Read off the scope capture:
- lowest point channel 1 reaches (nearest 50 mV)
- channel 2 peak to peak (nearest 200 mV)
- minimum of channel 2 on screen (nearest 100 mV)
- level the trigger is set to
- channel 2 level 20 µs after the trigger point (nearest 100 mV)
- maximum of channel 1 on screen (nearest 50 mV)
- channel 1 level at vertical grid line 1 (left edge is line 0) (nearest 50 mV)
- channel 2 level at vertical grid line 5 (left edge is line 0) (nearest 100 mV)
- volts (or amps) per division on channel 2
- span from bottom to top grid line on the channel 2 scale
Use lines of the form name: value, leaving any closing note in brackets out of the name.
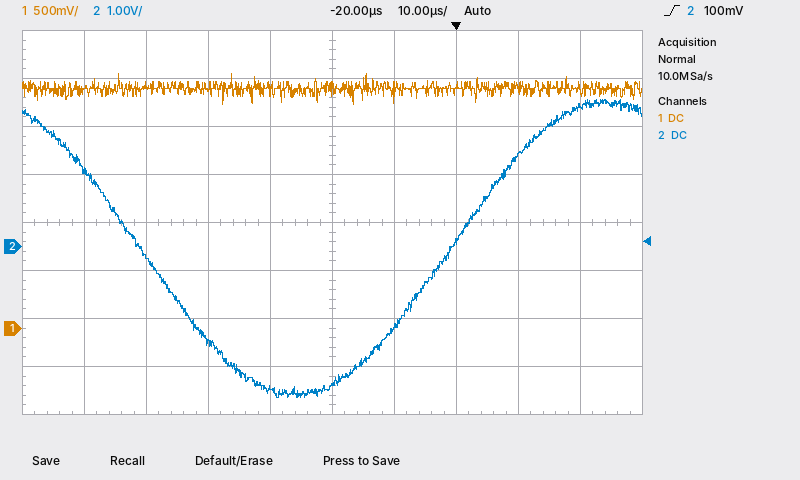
lowest point channel 1 reaches: 2.35 V
channel 2 peak to peak: 6.2 V
minimum of channel 2 on screen: -3.1 V
level the trigger is set to: 100 mV
channel 2 level 20 µs after the trigger point: 2.9 V
maximum of channel 1 on screen: 2.65 V
channel 1 level at vertical grid line 1 (left edge is line 0): 2.50 V
channel 2 level at vertical grid line 5 (left edge is line 0): -2.9 V
volts (or amps) per division on channel 2: 1 V
span from bottom to top grid line on the channel 2 scale: 8 V
